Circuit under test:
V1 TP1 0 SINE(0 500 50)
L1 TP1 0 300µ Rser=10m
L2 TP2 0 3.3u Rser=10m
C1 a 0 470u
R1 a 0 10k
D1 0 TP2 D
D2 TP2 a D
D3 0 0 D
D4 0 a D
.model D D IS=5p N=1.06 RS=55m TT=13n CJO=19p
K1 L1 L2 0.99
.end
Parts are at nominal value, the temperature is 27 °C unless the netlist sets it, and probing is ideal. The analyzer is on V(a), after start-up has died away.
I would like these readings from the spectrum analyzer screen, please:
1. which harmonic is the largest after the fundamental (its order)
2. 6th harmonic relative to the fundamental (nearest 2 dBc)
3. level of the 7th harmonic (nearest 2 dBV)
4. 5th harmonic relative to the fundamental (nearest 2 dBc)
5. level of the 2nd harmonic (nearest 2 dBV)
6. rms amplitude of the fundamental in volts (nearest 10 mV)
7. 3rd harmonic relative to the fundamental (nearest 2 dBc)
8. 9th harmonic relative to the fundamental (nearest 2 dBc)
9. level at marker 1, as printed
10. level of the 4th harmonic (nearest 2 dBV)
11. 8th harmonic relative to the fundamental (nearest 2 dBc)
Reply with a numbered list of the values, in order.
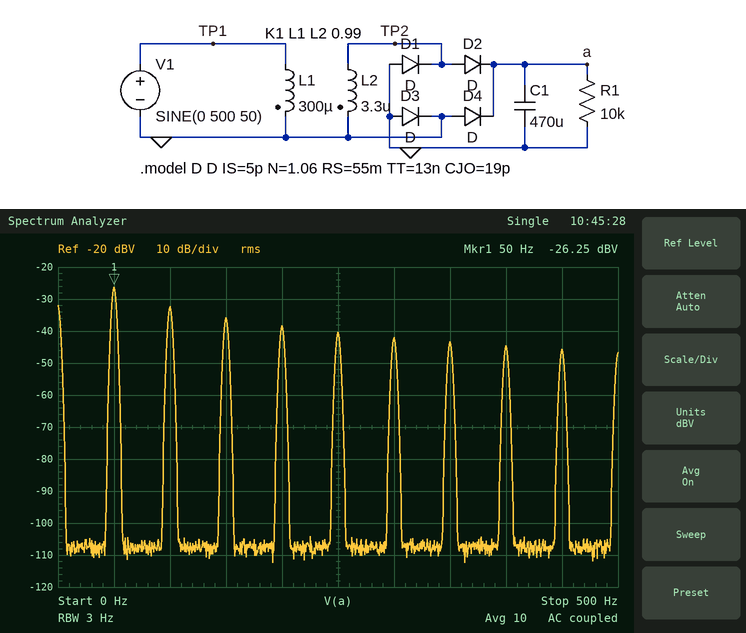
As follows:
1. 2
2. -16 dBc
3. -44 dBV
4. -14 dBc
5. -32 dBV
6. 50 mV
7. -10 dBc
8. -20 dBc
9. -26.25 dBV
10. -38 dBV
11. -18 dBc
